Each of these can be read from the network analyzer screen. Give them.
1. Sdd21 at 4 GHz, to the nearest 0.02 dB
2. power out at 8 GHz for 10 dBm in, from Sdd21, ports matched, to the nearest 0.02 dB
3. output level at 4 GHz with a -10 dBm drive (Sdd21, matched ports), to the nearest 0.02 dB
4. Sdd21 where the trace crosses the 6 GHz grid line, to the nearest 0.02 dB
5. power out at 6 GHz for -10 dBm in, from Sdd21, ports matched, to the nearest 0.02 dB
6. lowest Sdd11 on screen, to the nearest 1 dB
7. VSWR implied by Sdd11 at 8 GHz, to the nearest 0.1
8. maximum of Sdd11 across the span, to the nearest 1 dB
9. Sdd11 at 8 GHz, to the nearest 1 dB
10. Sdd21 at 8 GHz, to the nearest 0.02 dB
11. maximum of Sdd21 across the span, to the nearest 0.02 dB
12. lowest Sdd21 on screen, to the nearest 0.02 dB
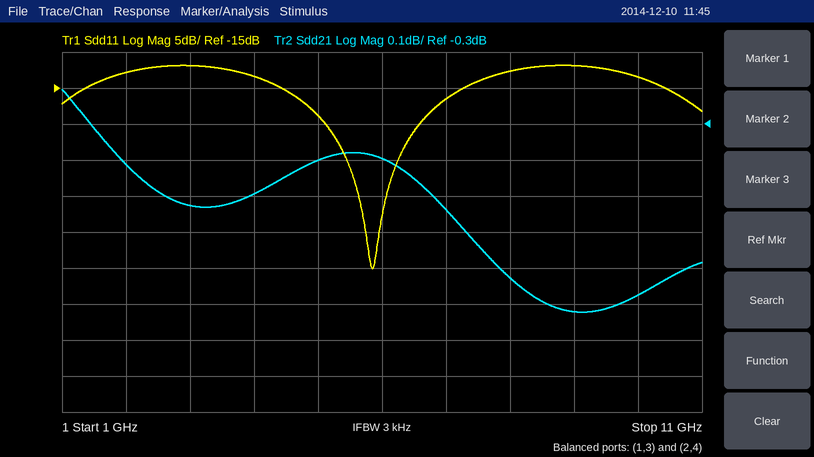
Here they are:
-0.50 dB
9.28 dBm
-10.50 dBm
-0.40 dB
-10.40 dBm
-40 dB
1.6
-12 dB
-13 dB
-0.72 dB
-0.20 dB
-0.82 dB
